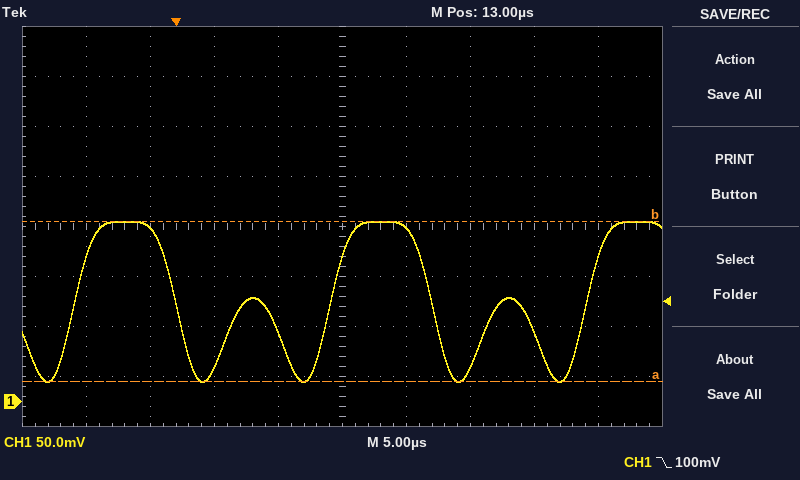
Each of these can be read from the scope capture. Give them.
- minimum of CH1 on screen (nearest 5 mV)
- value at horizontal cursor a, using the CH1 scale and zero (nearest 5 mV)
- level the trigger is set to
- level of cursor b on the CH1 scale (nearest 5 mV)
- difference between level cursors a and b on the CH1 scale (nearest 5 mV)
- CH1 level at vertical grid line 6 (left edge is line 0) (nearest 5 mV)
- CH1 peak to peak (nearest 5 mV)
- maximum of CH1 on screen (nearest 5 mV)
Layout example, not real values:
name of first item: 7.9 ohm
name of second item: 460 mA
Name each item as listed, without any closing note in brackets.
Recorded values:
minimum of CH1 on screen: 20 mV
value at horizontal cursor a, using the CH1 scale and zero: 20 mV
level the trigger is set to: 100 mV
level of cursor b on the CH1 scale: 180 mV
difference between level cursors a and b on the CH1 scale: 160 mV
CH1 level at vertical grid line 6 (left edge is line 0): 175 mV
CH1 peak to peak: 160 mV
maximum of CH1 on screen: 180 mV
